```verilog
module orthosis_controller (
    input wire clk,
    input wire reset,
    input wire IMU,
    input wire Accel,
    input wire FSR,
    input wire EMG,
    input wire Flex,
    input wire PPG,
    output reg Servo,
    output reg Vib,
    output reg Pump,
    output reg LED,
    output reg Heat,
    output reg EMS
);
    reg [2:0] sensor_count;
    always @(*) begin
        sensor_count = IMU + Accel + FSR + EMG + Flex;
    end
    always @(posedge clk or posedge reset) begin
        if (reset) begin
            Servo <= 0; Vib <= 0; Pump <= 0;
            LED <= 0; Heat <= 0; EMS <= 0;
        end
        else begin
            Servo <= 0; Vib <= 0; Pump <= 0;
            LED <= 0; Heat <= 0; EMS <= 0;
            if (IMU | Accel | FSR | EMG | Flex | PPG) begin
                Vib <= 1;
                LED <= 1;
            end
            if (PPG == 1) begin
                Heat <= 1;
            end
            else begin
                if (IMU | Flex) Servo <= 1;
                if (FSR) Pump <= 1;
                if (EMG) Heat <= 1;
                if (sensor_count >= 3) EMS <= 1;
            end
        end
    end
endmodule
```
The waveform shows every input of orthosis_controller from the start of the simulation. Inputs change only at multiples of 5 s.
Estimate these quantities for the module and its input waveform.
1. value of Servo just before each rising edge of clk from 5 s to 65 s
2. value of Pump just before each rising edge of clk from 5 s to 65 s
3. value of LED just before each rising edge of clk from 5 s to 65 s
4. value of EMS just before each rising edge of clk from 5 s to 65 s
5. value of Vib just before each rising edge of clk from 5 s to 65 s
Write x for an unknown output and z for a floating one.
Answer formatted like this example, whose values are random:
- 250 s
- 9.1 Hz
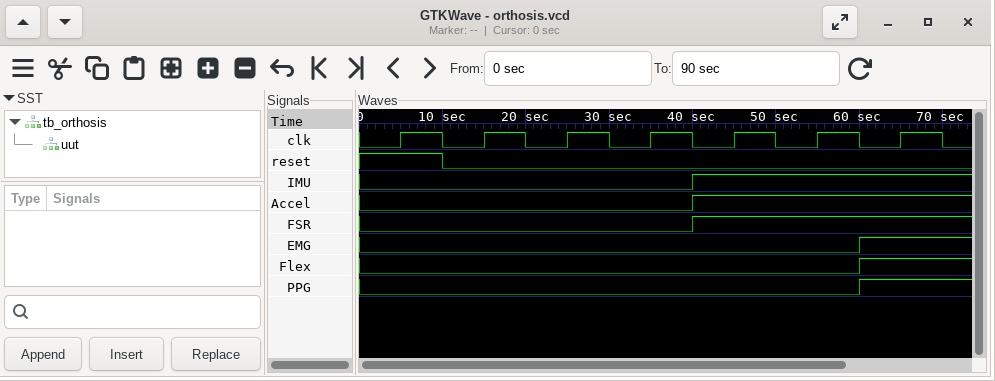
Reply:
- 0 0 0 0 0 1 1
- 0 0 0 0 0 1 1
- 0 0 0 0 0 1 1
- 0 0 0 0 0 1 1
- 0 0 0 0 0 1 1
